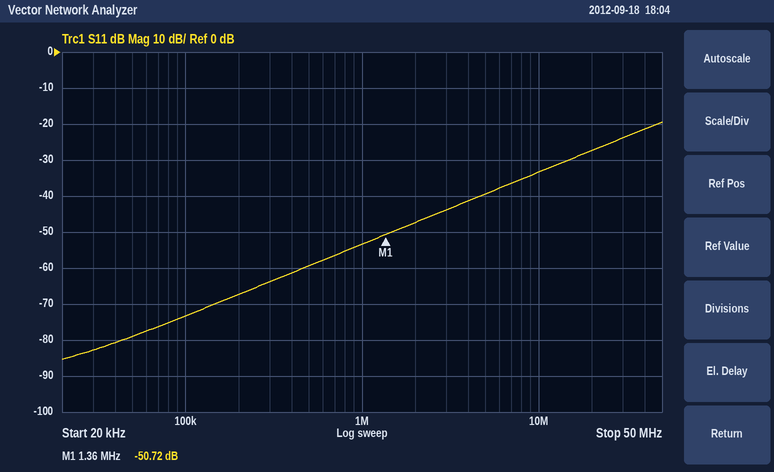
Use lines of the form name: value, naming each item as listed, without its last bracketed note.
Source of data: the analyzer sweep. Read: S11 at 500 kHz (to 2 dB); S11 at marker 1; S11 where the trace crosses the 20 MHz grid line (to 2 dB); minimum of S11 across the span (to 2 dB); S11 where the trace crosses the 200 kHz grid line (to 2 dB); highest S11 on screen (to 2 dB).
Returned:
S11 at 500 kHz: -60 dB
S11 at marker 1: -50.72 dB
S11 where the trace crosses the 20 MHz grid line: -28 dB
minimum of S11 across the span: -86 dB
S11 where the trace crosses the 200 kHz grid line: -68 dB
highest S11 on screen: -20 dB
